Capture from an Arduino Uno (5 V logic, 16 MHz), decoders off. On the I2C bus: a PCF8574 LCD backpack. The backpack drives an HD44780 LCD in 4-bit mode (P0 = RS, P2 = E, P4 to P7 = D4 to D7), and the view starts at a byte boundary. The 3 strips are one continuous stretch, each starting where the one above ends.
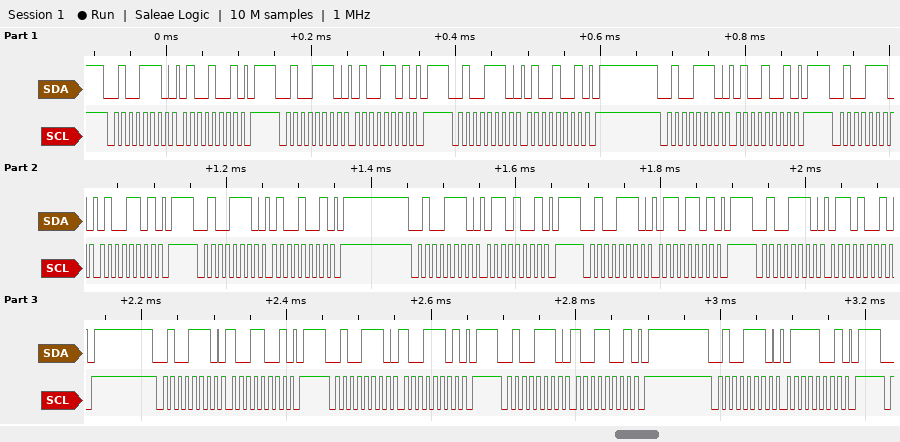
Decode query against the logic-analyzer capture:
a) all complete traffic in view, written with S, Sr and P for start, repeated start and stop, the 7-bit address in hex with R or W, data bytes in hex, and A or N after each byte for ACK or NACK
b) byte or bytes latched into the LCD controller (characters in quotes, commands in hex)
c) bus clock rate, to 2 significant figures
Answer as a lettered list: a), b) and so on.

a) S 27W A 49 A P S 27W A 4D A P S 27W A 49 A P S 27W A 49 A P S 27W A 4D A P S 27W A 49 A P S 27W A 69 A P S 27W A 6D A P S 27W A 69 A P S 27W A 99 A P S 27W A 9D A P S 27W A 99 A P S 27W A 79 A P
b) 'D' 'i'
c) 100 kHz
